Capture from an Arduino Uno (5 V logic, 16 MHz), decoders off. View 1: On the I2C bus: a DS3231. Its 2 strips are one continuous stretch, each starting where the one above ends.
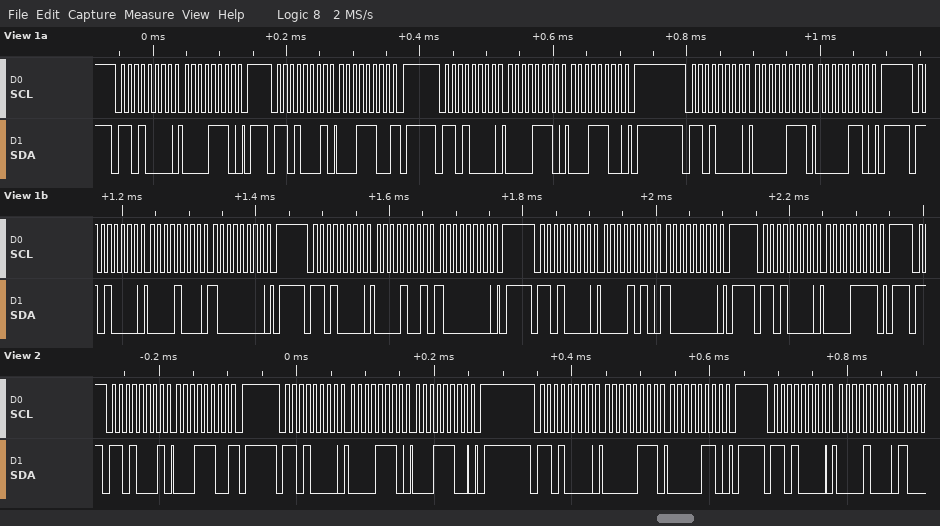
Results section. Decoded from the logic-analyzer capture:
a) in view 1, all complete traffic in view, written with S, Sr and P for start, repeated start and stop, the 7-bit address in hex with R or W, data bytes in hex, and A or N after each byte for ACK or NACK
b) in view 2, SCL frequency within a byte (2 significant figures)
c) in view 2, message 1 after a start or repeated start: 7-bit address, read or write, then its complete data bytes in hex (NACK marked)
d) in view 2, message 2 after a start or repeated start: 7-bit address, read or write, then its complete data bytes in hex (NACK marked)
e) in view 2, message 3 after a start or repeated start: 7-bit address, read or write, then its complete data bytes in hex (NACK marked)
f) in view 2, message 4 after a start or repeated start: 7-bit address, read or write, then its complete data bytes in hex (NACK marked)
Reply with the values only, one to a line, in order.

S 68W A 0E A P S 68R A 1C N P S 68W A 0E A 1C A P S 68W A 07 A 06 A P S 68W A 08 A 80 A P S 68W A 09 A 80 A P S 68W A 0A A 80 A P S 68W A 0F A P
100 kHz
0x68 read: 1C NACK
0x68 write: 0E 1C
0x68 write: 07 06
0x68 write: 08
